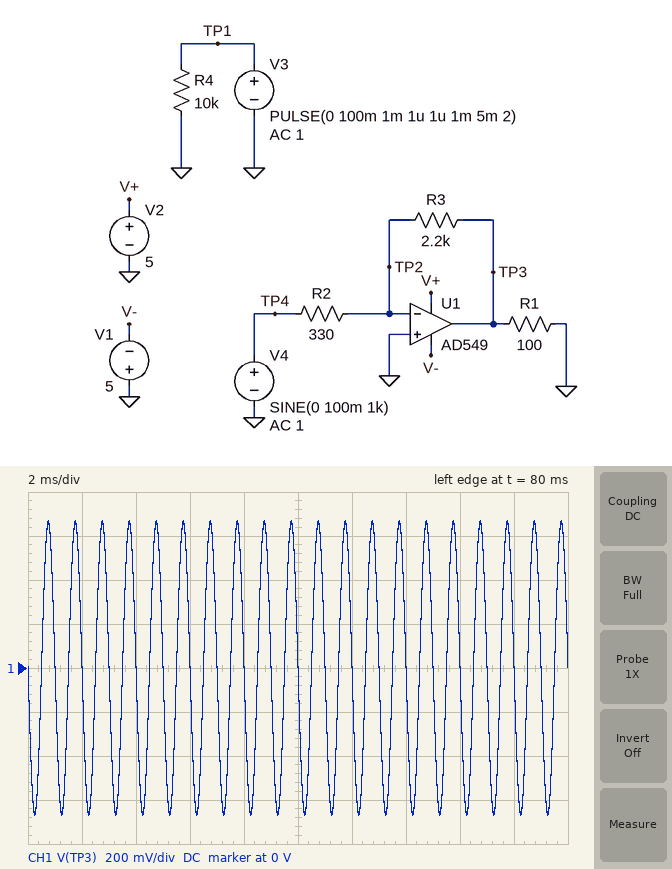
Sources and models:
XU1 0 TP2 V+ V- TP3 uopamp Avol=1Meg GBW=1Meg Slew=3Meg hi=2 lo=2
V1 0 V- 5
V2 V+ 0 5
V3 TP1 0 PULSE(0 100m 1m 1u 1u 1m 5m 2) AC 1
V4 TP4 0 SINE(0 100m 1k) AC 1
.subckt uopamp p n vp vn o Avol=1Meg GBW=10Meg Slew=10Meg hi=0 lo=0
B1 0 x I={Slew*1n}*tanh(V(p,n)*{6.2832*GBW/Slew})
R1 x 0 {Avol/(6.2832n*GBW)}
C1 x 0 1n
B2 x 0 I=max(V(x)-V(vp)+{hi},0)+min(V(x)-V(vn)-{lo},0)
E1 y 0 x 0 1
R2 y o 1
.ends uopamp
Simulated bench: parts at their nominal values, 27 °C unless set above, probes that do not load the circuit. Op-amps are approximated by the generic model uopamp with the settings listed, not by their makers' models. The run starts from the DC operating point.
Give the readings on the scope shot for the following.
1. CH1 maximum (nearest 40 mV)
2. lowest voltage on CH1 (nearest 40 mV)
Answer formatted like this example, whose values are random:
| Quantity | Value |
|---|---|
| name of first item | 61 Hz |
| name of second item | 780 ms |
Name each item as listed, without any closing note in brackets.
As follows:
| Quantity | Value |
|---|---|
| CH1 maximum | 680 mV |
| lowest voltage on CH1 | -680 mV |
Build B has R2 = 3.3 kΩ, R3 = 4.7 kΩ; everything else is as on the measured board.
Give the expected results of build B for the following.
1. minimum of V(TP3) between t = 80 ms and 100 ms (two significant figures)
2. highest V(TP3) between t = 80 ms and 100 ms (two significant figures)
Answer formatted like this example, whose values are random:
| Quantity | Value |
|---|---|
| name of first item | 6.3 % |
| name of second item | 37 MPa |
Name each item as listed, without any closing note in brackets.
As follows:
| Quantity | Value |
|---|---|
| minimum of V(TP3) between t = 80 ms and 100 ms | -140 mV |
| highest V(TP3) between t = 80 ms and 100 ms | 140 mV |
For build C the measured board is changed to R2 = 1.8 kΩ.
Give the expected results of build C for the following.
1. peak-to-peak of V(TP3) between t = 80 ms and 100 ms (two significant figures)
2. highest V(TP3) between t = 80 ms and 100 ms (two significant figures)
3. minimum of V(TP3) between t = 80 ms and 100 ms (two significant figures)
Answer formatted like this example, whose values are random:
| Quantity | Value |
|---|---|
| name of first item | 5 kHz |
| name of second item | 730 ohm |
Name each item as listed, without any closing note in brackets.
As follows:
| Quantity | Value |
|---|---|
| peak-to-peak of V(TP3) between t = 80 ms and 100 ms | 240 mV |
| highest V(TP3) between t = 80 ms and 100 ms | 120 mV |
| minimum of V(TP3) between t = 80 ms and 100 ms | -120 mV |
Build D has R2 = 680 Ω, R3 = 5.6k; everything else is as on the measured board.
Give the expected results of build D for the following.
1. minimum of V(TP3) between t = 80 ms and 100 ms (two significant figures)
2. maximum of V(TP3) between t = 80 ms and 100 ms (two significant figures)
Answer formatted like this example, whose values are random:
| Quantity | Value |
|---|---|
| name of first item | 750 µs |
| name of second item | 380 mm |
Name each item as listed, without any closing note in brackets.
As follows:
| Quantity | Value |
|---|---|
| minimum of V(TP3) between t = 80 ms and 100 ms | -820 mV |
| maximum of V(TP3) between t = 80 ms and 100 ms | 820 mV |
